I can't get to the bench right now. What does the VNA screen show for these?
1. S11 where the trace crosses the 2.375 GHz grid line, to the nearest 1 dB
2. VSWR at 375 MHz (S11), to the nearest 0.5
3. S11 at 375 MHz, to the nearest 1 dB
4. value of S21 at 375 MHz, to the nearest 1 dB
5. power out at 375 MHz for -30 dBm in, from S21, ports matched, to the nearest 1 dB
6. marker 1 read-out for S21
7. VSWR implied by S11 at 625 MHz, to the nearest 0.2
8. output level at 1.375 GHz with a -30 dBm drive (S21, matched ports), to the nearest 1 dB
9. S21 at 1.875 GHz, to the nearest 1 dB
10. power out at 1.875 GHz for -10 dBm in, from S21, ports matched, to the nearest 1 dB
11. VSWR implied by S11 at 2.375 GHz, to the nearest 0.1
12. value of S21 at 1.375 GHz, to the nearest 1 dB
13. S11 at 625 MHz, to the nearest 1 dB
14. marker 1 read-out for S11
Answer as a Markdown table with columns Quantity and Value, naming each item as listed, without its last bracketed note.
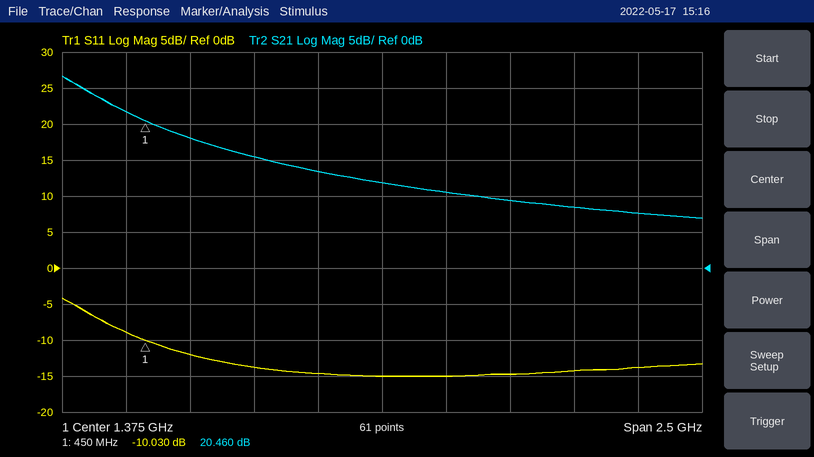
| Quantity | Value |
|---|---|
| S11 where the trace crosses the 2.375 GHz grid line, to the nearest 1 dB | -14 dB |
| VSWR at 375 MHz (S11), to the nearest 0.5 | 2.0 |
| S11 at 375 MHz, to the nearest 1 dB | -9 dB |
| value of S21 at 375 MHz, to the nearest 1 dB | 22 dB |
| power out at 375 MHz for -30 dBm in, from S21, ports matched, to the nearest 1 dB | -8 dBm |
| marker 1 read-out for S21 | 20.460 dB |
| VSWR implied by S11 at 625 MHz, to the nearest 0.2 | 1.6 |
| output level at 1.375 GHz with a -30 dBm drive (S21, matched ports), to the nearest 1 dB | -18 dBm |
| S21 at 1.875 GHz, to the nearest 1 dB | 9 dB |
| power out at 1.875 GHz for -10 dBm in, from S21, ports matched, to the nearest 1 dB | -1 dBm |
| VSWR implied by S11 at 2.375 GHz, to the nearest 0.1 | 1.5 |
| value of S21 at 1.375 GHz, to the nearest 1 dB | 12 dB |
| S11 at 625 MHz, to the nearest 1 dB | -12 dB |
| marker 1 read-out for S11 | -10.030 dB |
